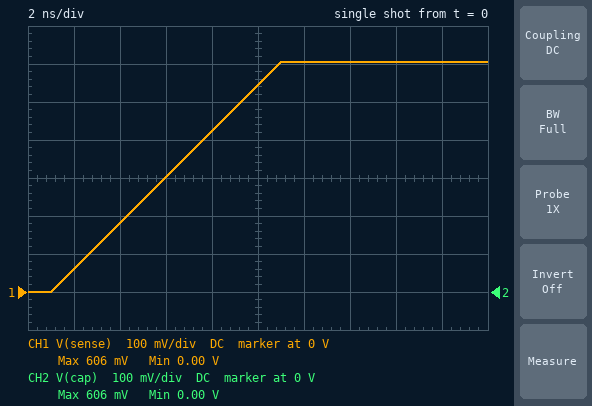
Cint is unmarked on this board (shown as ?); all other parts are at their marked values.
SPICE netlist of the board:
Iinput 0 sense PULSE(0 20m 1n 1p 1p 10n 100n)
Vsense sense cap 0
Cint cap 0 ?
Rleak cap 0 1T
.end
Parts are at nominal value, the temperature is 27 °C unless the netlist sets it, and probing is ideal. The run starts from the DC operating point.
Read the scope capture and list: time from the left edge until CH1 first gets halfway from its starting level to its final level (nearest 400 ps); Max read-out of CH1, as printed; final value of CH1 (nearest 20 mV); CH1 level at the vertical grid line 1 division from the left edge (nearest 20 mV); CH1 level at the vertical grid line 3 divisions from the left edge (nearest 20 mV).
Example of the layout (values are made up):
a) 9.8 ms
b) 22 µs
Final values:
a) 6.0 ns
b) 606 mV
c) 600 mV
d) 60 mV
e) 300 mV
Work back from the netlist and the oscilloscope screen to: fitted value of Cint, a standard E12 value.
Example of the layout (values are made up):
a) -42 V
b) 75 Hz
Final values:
a) 330 pF
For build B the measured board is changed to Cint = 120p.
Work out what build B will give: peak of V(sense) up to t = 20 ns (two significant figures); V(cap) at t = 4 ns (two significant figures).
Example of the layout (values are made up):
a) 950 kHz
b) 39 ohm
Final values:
a) 1.7 V
b) 500 mV
